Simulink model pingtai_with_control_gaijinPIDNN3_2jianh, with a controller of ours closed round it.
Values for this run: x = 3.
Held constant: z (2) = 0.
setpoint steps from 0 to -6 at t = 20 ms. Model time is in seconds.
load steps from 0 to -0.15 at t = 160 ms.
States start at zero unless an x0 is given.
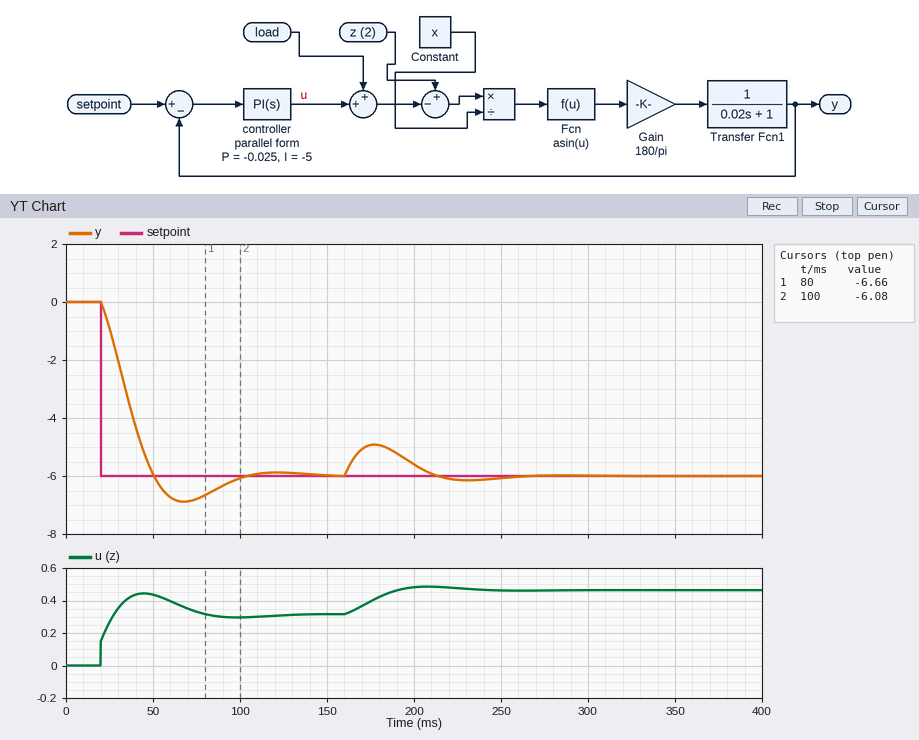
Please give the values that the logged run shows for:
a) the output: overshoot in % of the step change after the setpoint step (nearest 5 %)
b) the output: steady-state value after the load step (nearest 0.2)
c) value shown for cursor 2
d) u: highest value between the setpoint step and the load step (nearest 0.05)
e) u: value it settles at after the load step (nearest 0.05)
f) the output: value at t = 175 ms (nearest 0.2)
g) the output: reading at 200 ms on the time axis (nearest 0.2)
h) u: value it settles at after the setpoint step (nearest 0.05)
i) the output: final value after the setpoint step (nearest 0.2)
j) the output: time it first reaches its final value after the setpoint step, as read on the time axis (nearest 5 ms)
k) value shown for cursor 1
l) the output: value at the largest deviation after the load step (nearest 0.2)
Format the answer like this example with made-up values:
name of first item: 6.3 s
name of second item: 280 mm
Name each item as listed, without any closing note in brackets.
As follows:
the output: overshoot in % of the step change after the setpoint step: 15 %
the output: steady-state value after the load step: -6.0
value shown for cursor 2: -6.08
u: highest value between the setpoint step and the load step: 0.45
u: value it settles at after the load step: 0.45
the output: value at t = 175 ms: -5.0
the output: reading at 200 ms on the time axis: -5.6
u: value it settles at after the setpoint step: 0.30
the output: final value after the setpoint step: -6.0
the output: time it first reaches its final value after the setpoint step, as read on the time axis: 50 ms
value shown for cursor 1: -6.66
the output: value at the largest deviation after the load step: -5.0
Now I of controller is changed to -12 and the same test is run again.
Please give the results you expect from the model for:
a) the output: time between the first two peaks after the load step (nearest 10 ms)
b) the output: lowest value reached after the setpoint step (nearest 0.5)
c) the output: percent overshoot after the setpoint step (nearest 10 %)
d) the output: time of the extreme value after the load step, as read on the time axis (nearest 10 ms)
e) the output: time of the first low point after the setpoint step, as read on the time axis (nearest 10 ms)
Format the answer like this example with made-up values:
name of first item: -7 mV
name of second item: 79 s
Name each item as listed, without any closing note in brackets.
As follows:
the output: time between the first two peaks after the load step: 60 ms
the output: lowest value reached after the setpoint step: -8.0
the output: percent overshoot after the setpoint step: 30 %
the output: time of the extreme value after the load step, as read on the time axis: 170 ms
the output: time of the first low point after the setpoint step, as read on the time axis: 50 ms
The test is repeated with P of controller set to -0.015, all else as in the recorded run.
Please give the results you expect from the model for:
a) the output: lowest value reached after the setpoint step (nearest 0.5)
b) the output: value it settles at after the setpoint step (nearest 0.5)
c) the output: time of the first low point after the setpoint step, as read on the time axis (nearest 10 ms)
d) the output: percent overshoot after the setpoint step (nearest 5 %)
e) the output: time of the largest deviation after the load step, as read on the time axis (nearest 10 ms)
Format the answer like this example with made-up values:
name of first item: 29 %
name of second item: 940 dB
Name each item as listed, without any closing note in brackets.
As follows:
the output: lowest value reached after the setpoint step: -7.0
the output: value it settles at after the setpoint step: -6.0
the output: time of the first low point after the setpoint step, as read on the time axis: 70 ms
the output: percent overshoot after the setpoint step: 20 %
the output: time of the largest deviation after the load step, as read on the time axis: 180 ms
